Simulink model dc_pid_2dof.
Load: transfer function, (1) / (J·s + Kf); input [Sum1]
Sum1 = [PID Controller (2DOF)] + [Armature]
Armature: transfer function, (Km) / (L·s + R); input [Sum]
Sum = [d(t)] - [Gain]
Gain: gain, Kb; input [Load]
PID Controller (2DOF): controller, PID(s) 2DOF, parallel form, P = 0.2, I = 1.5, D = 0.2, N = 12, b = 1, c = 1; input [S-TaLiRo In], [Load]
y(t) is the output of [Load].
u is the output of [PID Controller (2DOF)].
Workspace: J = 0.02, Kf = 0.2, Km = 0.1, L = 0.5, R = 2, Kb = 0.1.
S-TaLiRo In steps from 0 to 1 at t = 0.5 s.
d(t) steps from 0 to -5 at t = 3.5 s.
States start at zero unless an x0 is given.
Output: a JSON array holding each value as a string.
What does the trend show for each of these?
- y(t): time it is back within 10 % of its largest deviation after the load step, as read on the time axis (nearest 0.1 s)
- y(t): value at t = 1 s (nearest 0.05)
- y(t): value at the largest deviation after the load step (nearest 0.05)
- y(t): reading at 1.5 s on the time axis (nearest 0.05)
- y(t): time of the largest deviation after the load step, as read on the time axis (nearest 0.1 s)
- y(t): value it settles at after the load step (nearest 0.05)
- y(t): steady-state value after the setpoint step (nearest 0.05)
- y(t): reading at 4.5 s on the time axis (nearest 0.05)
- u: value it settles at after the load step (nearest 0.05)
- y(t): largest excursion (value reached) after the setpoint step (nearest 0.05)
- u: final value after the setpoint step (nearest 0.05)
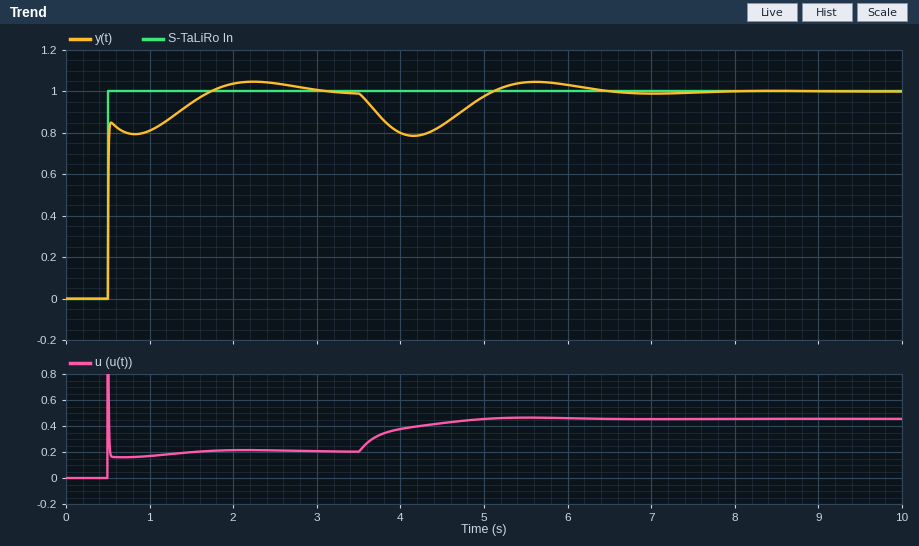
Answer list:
["6.2 s", "0.80", "0.80", "0.95", "4.2 s", "1.00", "1.00", "0.85", "0.45", "1.05", "0.20"]
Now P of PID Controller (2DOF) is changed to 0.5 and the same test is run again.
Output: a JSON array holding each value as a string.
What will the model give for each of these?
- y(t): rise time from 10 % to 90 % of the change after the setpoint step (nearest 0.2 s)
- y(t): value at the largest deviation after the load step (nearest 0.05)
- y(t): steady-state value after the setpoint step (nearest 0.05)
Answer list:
["0.8 s", "0.85", "1.00"]
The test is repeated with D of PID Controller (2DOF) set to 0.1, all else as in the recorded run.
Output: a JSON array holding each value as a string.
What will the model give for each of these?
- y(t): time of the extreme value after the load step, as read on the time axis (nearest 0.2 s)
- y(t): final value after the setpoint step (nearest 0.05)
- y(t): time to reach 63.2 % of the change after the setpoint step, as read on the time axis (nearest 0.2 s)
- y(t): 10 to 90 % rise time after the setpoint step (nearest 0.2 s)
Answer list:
["4.0 s", "1.00", "0.6 s", "0.6 s"]
